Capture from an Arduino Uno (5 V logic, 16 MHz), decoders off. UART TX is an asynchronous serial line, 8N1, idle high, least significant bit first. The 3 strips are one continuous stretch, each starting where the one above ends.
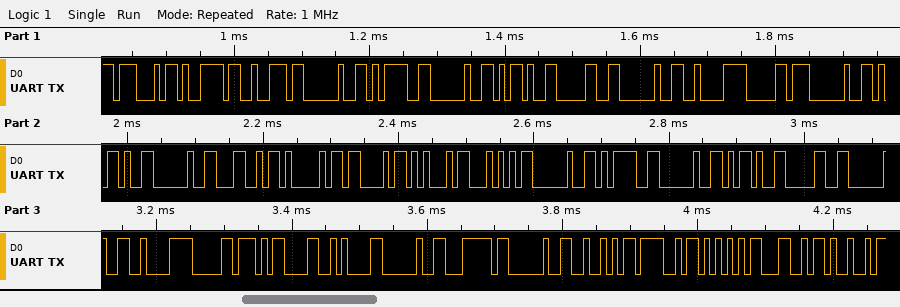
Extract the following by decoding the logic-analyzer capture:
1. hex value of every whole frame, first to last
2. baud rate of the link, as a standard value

47 79 72 20 3D 20 2D 30 20 C2 B0 20 2D 20 4C 41 43 45 54 20 3D 20 2D 30 20 C2 B0 0D 0A 20 7C 20 52 4F 55 4C 49
115200 baud
